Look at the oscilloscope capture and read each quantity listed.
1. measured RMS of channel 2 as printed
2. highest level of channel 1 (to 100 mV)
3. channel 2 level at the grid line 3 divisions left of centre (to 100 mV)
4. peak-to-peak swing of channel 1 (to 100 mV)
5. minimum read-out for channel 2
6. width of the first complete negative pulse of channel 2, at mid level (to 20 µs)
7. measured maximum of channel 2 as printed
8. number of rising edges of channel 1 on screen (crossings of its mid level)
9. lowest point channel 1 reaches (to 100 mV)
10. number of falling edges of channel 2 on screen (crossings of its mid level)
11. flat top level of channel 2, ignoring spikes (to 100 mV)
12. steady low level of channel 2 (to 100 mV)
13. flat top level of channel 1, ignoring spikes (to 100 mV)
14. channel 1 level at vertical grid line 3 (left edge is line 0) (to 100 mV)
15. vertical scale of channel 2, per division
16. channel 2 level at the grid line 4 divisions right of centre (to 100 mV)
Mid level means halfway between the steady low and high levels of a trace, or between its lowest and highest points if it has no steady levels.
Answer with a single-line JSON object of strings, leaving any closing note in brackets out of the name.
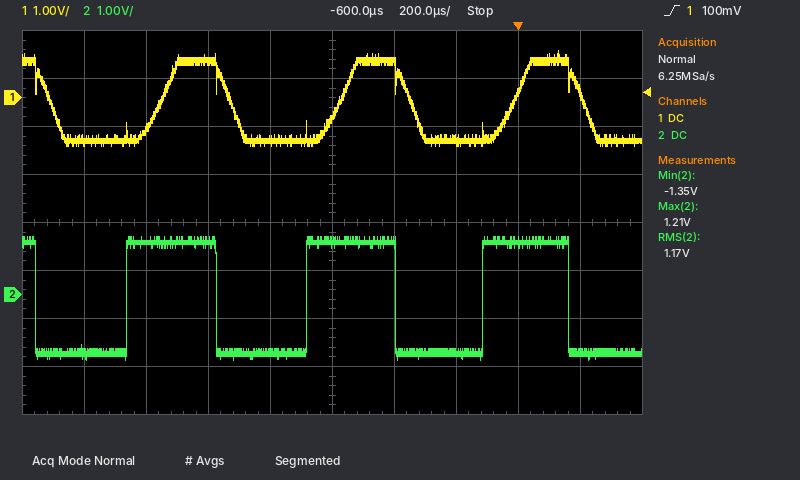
{"measured RMS of channel 2 as printed": "1.17 V", "highest level of channel 1": "1.0 V", "channel 2 level at the grid line 3 divisions left of centre": "1.1 V", "peak-to-peak swing of channel 1": "2.0 V", "minimum read-out for channel 2": "-1.35 V", "width of the first complete negative pulse of channel 2, at mid level": "300 µs", "measured maximum of channel 2 as printed": "1.21 V", "number of rising edges of channel 1 on screen": "3", "lowest point channel 1 reaches": "-1.0 V", "number of falling edges of channel 2 on screen": "4", "flat top level of channel 2, ignoring spikes": "1.1 V", "steady low level of channel 2": "-1.2 V", "flat top level of channel 1, ignoring spikes": "800 mV", "channel 1 level at vertical grid line 3 (left edge is line 0)": "800 mV", "vertical scale of channel 2, per division": "1 V", "channel 2 level at the grid line 4 divisions right of centre": "-1.2 V"}
